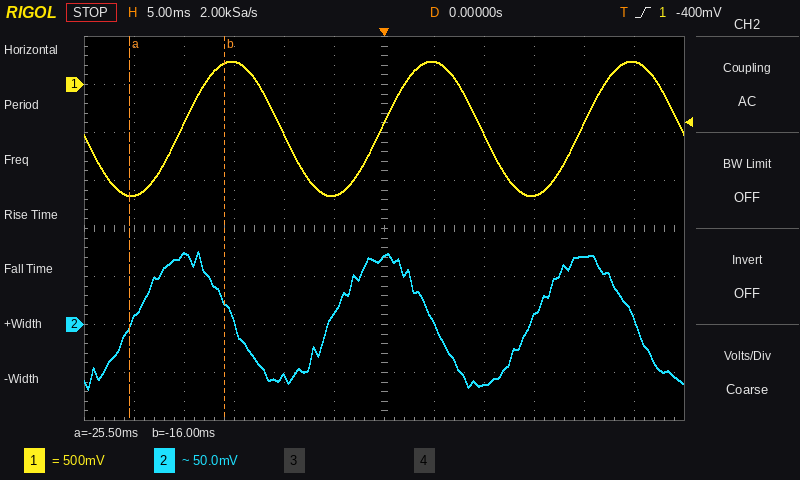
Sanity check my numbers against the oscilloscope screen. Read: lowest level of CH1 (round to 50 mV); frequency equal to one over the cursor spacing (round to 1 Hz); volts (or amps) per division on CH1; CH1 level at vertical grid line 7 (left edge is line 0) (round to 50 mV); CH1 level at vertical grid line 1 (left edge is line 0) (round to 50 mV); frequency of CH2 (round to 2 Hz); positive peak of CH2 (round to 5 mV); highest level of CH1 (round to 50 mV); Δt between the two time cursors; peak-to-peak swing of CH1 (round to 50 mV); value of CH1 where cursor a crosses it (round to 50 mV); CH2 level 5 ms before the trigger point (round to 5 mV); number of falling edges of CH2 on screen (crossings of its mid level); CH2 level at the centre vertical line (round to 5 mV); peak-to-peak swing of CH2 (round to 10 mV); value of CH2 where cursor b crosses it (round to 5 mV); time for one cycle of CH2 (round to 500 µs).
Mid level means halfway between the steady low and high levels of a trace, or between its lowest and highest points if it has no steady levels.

-1.15 V
105 Hz
500 mV
250 mV
-1.15 V
50 Hz
75 mV
250 mV
9.5 ms
1.40 V
-1.15 V
10 mV
3
70 mV
140 mV
25 mV
20.0 ms
